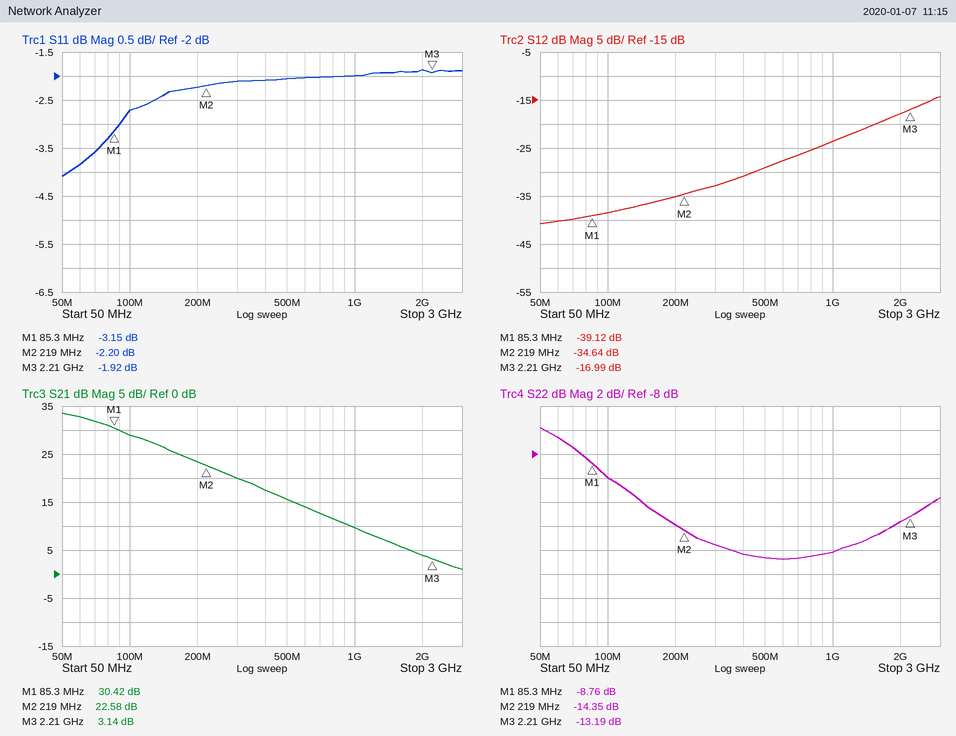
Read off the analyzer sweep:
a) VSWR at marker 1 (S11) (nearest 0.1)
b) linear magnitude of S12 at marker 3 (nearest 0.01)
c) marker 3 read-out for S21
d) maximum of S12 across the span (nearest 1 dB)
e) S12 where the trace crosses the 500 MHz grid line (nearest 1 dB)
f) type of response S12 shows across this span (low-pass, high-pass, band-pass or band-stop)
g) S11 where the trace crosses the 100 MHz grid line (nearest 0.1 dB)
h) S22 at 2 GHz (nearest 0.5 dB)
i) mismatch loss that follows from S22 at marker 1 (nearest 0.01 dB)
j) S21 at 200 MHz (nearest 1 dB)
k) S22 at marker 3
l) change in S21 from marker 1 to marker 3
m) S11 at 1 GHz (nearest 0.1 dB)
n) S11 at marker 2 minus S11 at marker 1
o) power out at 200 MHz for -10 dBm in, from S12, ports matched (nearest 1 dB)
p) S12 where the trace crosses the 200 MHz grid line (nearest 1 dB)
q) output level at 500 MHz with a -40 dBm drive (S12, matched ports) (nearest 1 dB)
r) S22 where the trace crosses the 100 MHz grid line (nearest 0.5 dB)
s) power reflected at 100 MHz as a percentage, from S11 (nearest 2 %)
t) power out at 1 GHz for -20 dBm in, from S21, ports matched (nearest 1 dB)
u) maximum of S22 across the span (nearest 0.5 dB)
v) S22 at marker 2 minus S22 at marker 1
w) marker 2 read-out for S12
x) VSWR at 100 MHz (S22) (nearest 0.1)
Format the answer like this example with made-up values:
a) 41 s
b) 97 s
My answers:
a) 5.6
b) 0.14
c) 3.14 dB
d) -14 dB
e) -29 dB
f) high-pass
g) -2.7 dB
h) -13.5 dB
i) 0.62 dB
j) 23 dB
k) -13.19 dB
l) -27.28 dB
m) -2.0 dB
n) 0.95 dB
o) -45 dBm
p) -35 dB
q) -69 dBm
r) -10.0 dB
s) 54 %
t) -10 dBm
u) -6.0 dB
v) -5.59 dB
w) -34.64 dB
x) 1.9
